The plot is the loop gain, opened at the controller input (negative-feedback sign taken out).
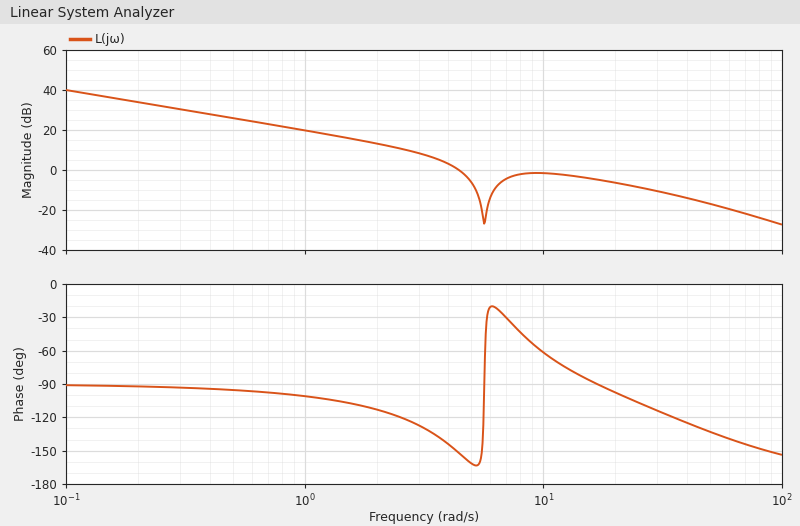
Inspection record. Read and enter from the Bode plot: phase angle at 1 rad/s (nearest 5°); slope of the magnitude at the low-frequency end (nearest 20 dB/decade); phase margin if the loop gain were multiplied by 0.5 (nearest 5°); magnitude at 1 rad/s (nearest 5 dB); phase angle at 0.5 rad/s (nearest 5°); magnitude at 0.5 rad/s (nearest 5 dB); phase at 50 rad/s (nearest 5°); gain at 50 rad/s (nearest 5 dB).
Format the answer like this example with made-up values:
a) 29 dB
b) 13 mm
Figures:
a) -100°
b) -20 dB/decade
c) 45°
d) 20 dB
e) -95°
f) 25 dB
g) -135°
h) -15 dB
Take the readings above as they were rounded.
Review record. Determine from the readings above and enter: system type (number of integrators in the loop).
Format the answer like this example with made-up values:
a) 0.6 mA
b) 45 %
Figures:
a) 1
